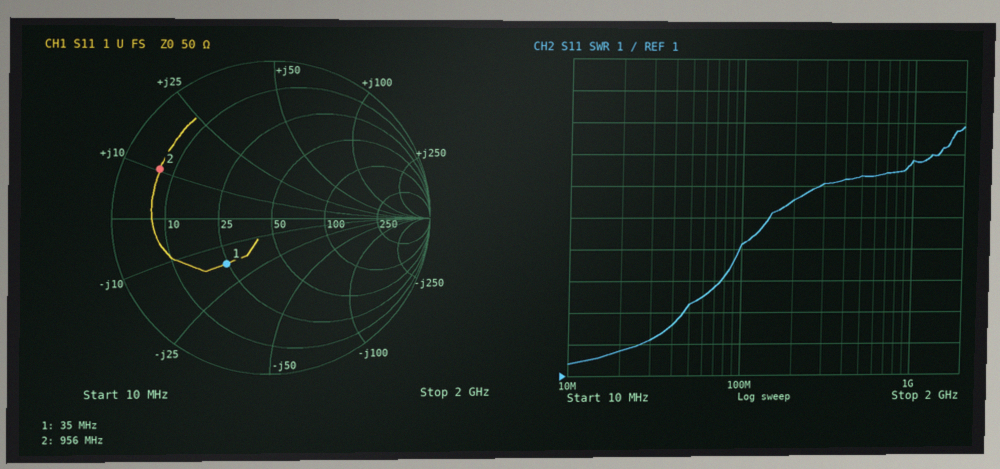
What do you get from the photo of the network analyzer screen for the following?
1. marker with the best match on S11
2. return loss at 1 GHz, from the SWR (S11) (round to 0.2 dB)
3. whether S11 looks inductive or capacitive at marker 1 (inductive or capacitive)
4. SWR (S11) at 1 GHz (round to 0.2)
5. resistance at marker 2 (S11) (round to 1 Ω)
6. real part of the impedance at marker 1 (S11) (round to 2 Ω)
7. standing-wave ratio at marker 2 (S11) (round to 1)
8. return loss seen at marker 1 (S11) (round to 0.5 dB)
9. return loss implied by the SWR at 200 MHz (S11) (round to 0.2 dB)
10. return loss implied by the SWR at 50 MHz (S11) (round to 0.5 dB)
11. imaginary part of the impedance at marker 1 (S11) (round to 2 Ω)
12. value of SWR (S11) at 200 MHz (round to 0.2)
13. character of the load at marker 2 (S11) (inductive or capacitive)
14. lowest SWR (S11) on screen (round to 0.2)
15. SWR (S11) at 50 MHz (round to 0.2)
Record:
marker 1
2.2 dB
capacitive
7.8
7 Ω
24 Ω
8
8.0 dB
2.6 dB
5.5 dB
-16 Ω
6.6
inductive
1.4
3.2
